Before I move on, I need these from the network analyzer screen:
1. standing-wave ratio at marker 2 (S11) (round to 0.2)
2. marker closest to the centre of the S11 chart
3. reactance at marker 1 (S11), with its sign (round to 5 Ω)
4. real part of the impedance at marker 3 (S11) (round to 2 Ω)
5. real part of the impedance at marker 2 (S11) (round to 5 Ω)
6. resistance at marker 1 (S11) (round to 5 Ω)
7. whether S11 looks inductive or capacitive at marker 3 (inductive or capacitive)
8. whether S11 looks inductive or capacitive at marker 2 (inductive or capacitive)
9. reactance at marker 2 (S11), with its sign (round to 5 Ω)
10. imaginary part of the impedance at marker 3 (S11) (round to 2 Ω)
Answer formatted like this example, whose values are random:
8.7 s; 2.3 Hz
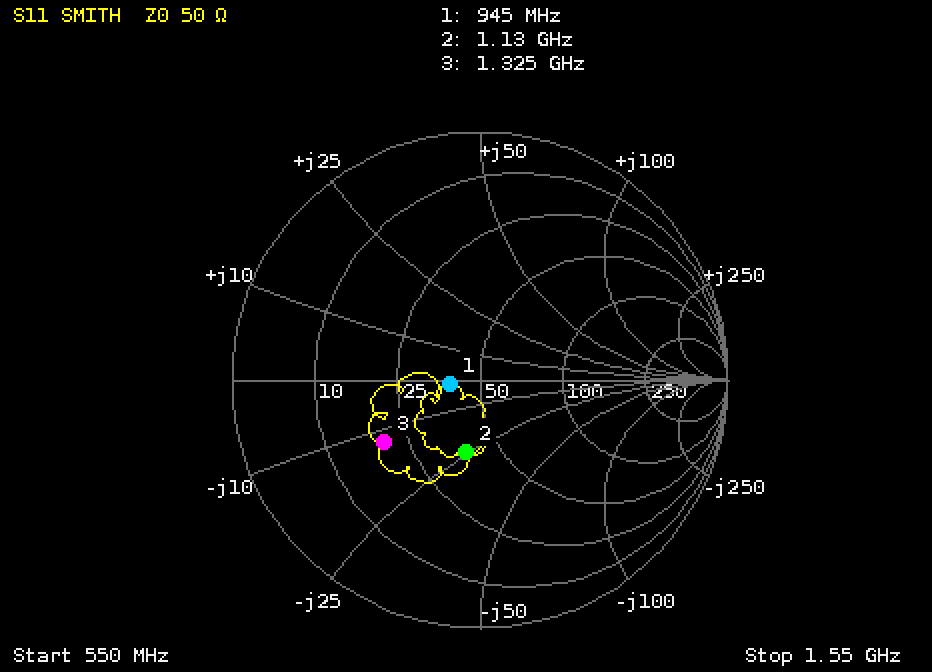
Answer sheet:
1.8; marker 1; 0 Ω; 20 Ω; 40 Ω; 40 Ω; capacitive; capacitive; -25 Ω; -12 Ω
